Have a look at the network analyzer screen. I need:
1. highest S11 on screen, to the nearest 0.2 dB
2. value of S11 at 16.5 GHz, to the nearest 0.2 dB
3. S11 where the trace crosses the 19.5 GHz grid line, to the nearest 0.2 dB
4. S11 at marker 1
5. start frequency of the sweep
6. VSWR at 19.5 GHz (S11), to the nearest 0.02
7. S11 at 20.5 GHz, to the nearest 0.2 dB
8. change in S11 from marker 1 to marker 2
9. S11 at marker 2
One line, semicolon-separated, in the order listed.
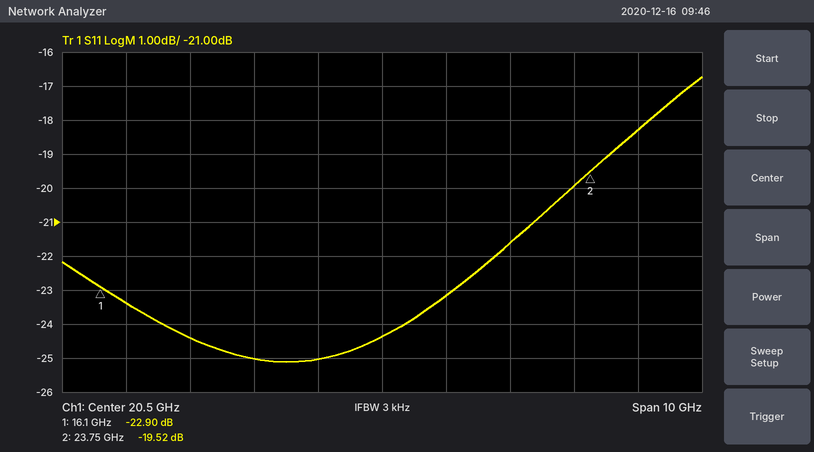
-16.8 dB; -23.4 dB; -25.0 dB; -22.90 dB; 15.5 GHz; 1.12; -24.4 dB; 3.38 dB; -19.52 dB
